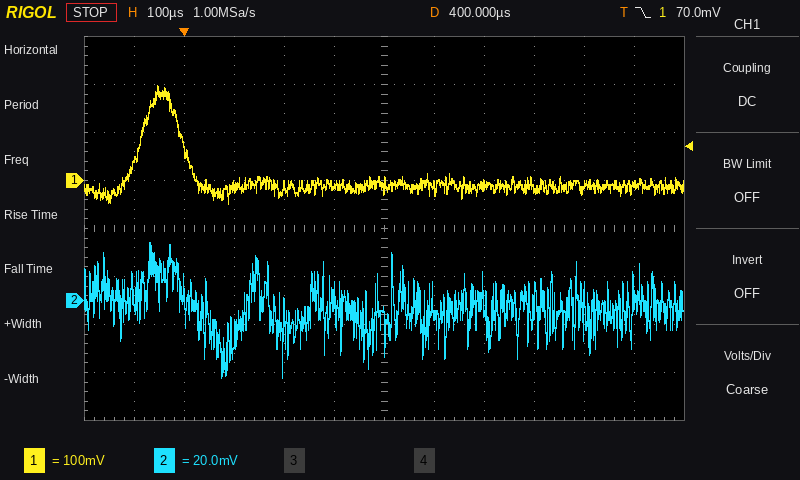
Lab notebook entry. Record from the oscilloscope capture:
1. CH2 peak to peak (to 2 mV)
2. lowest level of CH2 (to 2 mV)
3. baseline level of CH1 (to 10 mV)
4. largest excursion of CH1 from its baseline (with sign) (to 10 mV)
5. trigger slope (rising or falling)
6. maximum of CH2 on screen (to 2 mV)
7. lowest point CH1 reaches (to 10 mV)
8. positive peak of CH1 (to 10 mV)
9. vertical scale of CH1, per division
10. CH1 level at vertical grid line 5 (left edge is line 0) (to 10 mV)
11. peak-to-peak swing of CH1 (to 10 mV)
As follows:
56 mV
-32 mV
-10 mV
+210 mV
falling
24 mV
-50 mV
200 mV
100 mV
-10 mV
250 mV
